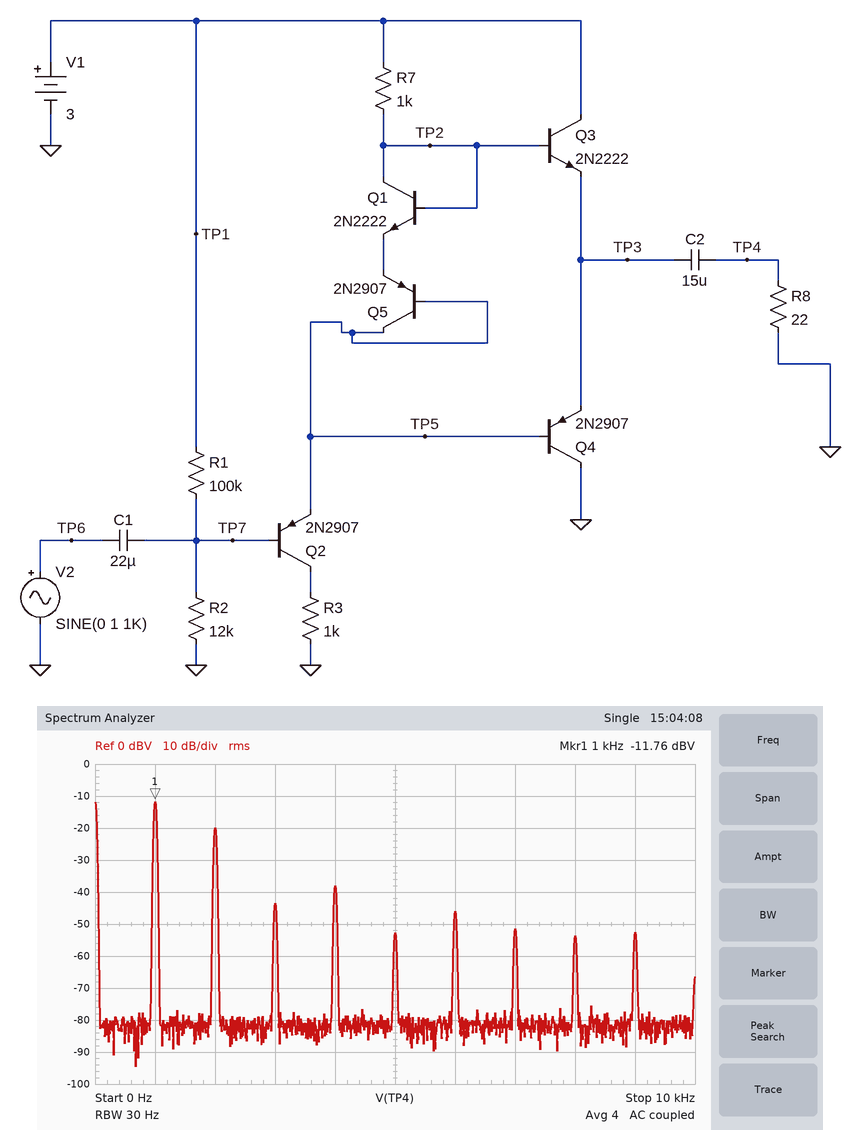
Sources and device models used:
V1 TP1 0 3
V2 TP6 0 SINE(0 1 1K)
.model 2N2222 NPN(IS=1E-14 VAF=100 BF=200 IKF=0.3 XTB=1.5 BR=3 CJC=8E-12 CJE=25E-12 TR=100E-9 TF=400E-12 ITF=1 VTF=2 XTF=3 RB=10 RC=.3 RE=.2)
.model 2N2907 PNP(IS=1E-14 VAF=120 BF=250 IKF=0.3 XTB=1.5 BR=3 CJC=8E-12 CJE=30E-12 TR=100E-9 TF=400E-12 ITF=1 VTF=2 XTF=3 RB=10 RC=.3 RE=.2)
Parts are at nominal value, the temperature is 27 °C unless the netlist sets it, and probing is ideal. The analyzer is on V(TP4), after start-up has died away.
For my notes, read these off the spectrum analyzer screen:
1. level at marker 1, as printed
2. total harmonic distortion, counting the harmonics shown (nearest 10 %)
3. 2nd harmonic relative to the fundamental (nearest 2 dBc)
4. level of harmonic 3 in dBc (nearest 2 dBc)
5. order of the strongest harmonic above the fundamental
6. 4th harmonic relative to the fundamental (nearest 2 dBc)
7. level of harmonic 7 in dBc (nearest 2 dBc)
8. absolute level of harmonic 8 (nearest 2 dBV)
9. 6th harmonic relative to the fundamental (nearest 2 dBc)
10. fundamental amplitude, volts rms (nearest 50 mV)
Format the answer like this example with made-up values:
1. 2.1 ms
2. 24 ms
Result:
1. -11.76 dBV
2. 40 %
3. -8 dBc
4. -32 dBc
5. 2
6. -26 dBc
7. -40 dBc
8. -54 dBV
9. -34 dBc
10. 250 mV
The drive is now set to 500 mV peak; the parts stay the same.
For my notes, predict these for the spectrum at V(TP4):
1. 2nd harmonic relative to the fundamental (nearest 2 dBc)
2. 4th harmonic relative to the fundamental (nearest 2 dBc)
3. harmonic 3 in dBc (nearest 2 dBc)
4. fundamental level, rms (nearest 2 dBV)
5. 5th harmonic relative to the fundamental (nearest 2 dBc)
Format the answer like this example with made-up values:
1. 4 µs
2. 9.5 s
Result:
1. -22 dBc
2. -44 dBc
3. -28 dBc
4. -14 dBV
5. -34 dBc
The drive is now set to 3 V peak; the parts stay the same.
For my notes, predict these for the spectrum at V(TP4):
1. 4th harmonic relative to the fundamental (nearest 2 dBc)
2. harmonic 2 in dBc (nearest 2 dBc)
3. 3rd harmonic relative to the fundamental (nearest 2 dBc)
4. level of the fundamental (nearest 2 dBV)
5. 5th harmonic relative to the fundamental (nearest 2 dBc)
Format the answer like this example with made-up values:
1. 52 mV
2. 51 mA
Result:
1. -22 dBc
2. -2 dBc
3. -8 dBc
4. -10 dBV
5. -24 dBc
